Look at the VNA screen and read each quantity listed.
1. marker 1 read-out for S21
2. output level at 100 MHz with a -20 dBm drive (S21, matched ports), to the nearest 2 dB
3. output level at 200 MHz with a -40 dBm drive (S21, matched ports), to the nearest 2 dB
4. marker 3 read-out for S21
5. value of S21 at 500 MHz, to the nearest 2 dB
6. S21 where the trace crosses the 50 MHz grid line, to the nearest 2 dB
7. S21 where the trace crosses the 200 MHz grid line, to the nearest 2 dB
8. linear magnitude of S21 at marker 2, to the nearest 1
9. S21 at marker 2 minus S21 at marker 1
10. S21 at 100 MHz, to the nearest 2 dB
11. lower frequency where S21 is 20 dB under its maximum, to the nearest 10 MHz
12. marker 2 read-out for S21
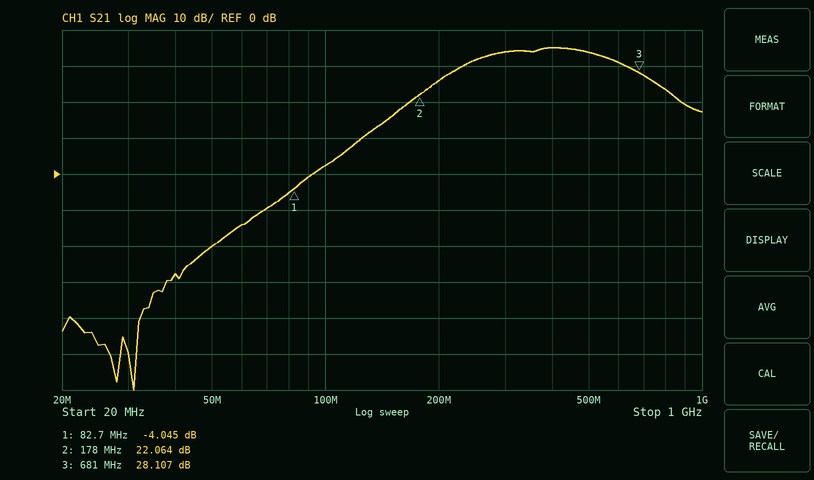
-4.045 dB
-18 dBm
-14 dBm
28.107 dB
34 dB
-20 dB
26 dB
13
26.109 dB
2 dB
150 MHz
22.064 dB
